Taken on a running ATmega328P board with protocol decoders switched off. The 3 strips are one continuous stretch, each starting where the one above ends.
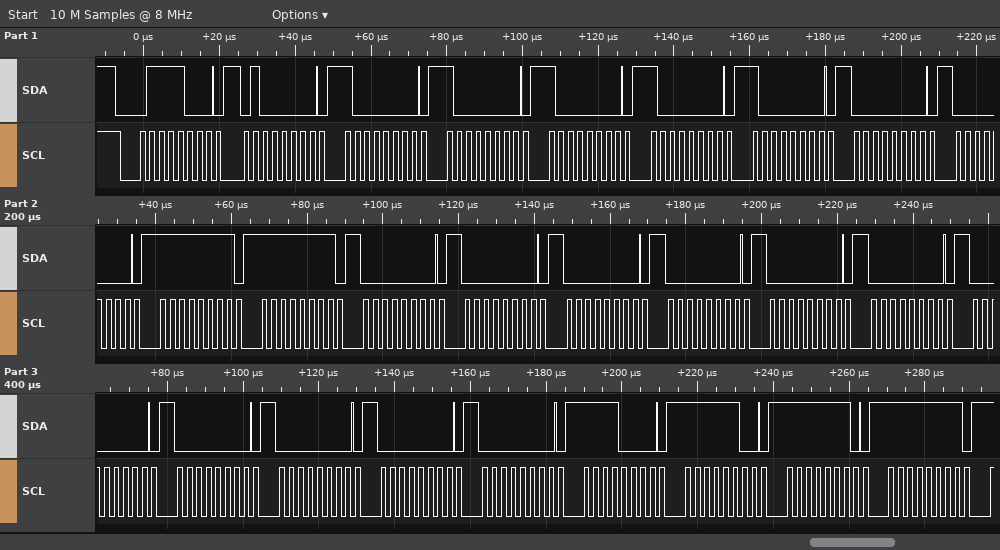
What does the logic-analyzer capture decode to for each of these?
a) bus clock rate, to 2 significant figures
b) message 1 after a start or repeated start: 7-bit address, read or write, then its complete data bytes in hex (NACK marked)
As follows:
400 kHz
0x3C write: 40 80 80 80 80 80 00 00 FF FF 00 00 00 00 00 00 00 00 00 00 00 F0 FC FE FF
